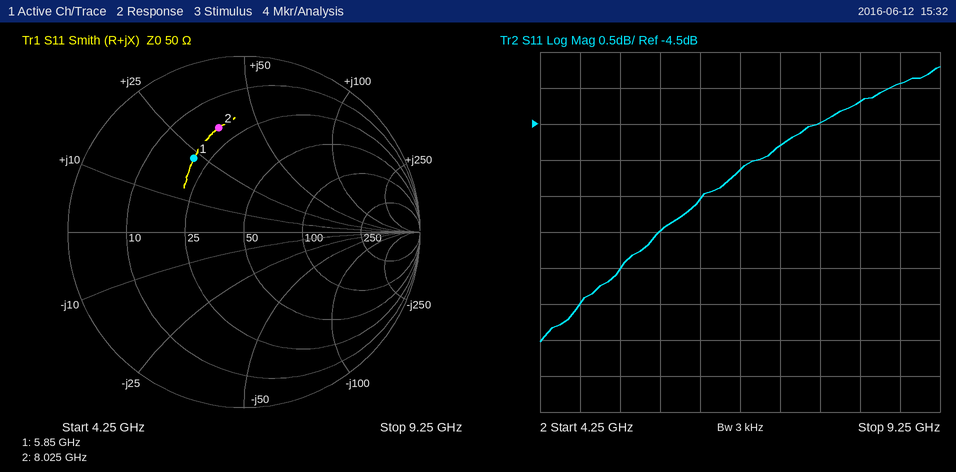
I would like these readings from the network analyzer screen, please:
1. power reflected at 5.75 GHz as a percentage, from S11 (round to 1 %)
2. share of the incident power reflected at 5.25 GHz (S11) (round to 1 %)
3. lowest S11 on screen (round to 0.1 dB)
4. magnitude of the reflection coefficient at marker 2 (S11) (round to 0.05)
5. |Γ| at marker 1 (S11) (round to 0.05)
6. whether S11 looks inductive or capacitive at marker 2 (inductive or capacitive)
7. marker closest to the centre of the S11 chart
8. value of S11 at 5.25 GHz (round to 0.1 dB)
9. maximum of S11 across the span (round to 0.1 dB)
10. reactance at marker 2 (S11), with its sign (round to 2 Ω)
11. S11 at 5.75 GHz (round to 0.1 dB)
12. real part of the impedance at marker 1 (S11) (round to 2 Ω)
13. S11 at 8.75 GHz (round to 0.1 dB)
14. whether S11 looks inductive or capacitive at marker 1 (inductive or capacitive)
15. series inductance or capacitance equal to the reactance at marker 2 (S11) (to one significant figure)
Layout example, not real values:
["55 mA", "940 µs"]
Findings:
["25 %", "22 %", "-7.5 dB", "0.60", "0.50", "inductive", "marker 1", "-6.5 dB", "-3.7 dB", "+36 Ω", "-6.0 dB", "20 Ω", "-3.9 dB", "inductive", "700 pH"]
